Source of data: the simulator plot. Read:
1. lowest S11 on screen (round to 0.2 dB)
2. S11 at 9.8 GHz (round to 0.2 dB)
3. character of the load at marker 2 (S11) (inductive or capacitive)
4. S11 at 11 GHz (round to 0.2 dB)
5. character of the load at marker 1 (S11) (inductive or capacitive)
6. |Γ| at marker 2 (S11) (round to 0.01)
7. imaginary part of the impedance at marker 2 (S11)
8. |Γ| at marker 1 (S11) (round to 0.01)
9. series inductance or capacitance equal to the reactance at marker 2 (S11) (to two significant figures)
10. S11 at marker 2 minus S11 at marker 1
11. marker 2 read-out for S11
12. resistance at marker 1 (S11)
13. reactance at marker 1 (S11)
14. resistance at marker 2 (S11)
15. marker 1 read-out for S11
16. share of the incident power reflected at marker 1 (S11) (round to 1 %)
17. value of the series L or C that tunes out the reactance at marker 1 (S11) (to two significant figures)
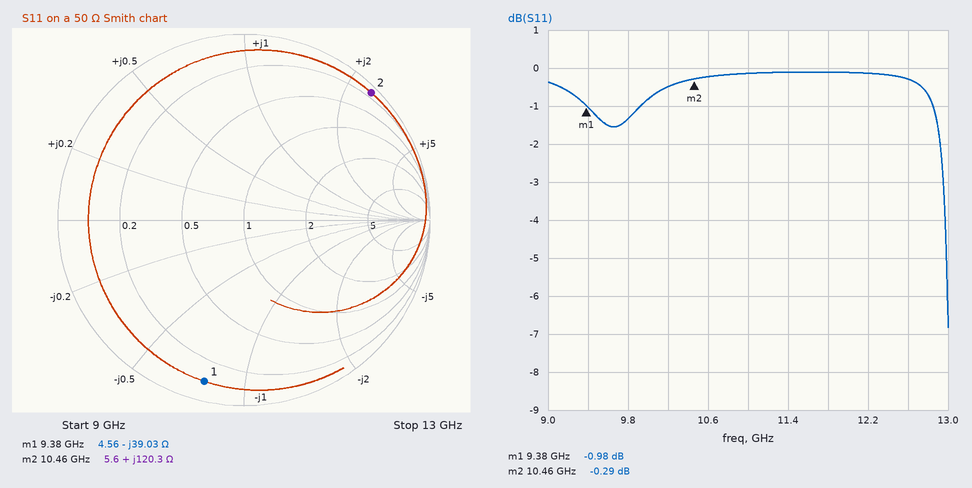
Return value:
-6.8 dB
-1.4 dB
inductive
-0.2 dB
capacitive
0.97
+120.3 Ω
0.89
1.8 nH
0.69 dB
-0.29 dB
4.56 Ω
-39.03 Ω
5.6 Ω
-0.98 dB
80 %
660 pH
